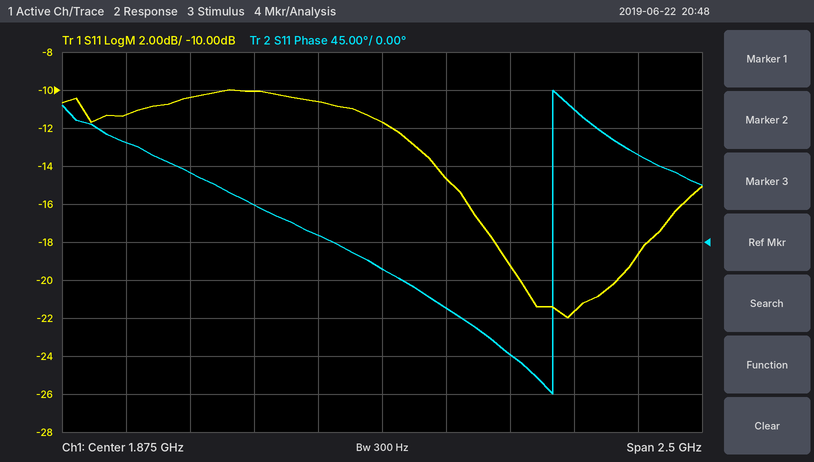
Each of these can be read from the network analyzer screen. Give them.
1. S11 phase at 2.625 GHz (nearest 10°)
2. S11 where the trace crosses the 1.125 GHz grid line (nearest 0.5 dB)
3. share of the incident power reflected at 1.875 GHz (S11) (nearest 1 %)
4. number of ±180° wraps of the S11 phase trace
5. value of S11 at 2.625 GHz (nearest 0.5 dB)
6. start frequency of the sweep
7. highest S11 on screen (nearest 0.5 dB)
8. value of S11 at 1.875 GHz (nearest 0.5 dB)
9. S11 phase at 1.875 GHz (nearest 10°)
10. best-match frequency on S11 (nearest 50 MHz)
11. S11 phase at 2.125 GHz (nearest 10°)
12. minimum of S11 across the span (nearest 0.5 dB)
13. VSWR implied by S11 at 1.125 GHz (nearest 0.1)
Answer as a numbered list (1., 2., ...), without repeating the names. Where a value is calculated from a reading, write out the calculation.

1. 160°
2. -10.5 dB
3. 10^(-11.5/10) ≈ 7 %
4. 1
5. -21.5 dB
6. 625 MHz
7. -10.0 dB
8. -11.5 dB
9. -30°
10. 2.60 GHz
11. -80°
12. -22.0 dB
13. |Γ| = 10^(-10.5/20) = 0.2985; VSWR = (1 + 0.2985)/(1 − 0.2985) ≈ 1.9
